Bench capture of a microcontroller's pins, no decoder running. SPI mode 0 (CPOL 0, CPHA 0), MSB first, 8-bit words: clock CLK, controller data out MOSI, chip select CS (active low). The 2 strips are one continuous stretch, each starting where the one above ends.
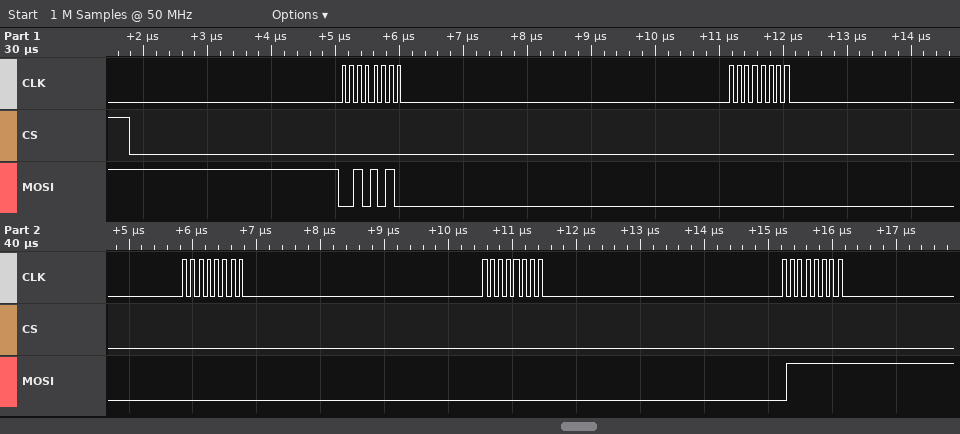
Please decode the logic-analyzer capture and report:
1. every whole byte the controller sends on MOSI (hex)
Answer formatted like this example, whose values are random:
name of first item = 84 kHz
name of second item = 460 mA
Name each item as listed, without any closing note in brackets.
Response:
every whole byte the controller sends on MOSI = 2A 00 00 00 7F
